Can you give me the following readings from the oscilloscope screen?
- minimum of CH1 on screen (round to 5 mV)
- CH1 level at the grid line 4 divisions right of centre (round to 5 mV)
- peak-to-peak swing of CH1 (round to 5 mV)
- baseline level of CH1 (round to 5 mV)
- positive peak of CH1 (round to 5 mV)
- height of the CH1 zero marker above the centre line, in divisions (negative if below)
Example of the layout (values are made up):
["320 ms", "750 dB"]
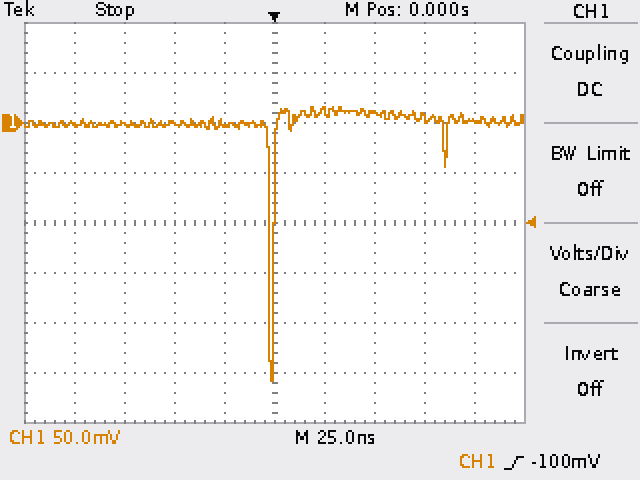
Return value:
["-260 mV", "0 mV", "275 mV", "0 mV", "15 mV", "+2.0 div"]
